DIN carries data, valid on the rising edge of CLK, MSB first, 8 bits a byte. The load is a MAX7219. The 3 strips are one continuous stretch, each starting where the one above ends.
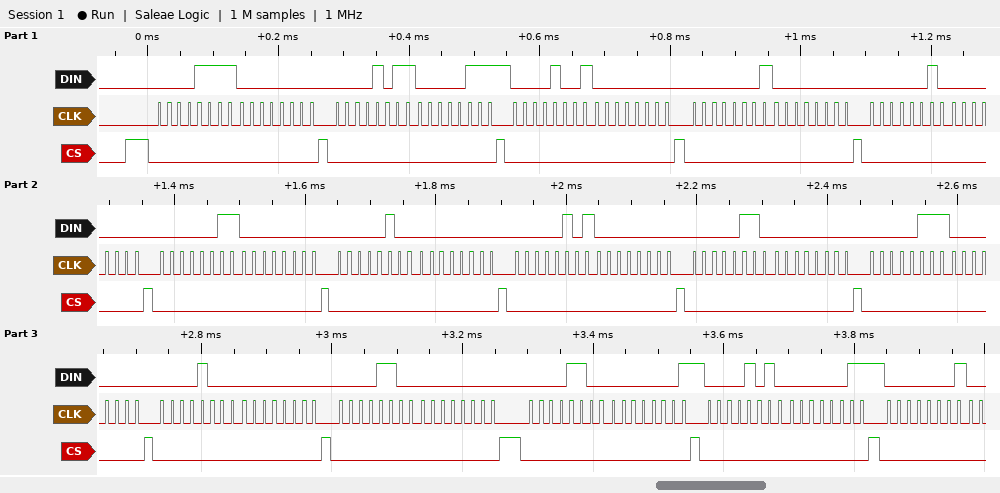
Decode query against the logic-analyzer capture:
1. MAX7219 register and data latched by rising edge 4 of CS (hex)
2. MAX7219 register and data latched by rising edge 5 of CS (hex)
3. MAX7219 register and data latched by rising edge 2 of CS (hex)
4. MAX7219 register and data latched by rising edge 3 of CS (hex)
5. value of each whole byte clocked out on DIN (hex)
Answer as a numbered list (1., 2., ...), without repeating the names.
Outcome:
1. register 0x9, data 0x00
2. register 0x1, data 0x00
3. register 0xF, data 0x00
4. register 0xB, data 0x07
5. 0F 00 0B 07 09 00 01 00 02 00 03 00 04 00 05 00 06 00 07 00 08 00 0C 00 0C 01 0A 03 01
